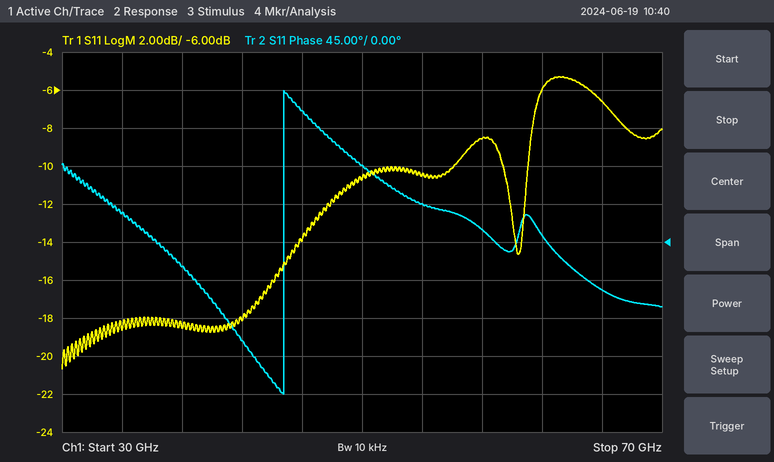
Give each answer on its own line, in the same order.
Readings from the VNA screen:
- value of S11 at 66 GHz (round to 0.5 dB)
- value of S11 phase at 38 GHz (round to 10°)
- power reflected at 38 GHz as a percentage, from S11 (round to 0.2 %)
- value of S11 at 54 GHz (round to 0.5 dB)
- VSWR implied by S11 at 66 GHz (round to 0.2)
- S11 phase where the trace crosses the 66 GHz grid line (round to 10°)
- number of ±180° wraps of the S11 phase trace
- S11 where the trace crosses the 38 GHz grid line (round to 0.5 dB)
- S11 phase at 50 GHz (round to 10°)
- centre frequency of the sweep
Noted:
-6.5 dB
-30°
1.4 %
-10.5 dB
2.8
-60°
1
-18.5 dB
90°
50 GHz
